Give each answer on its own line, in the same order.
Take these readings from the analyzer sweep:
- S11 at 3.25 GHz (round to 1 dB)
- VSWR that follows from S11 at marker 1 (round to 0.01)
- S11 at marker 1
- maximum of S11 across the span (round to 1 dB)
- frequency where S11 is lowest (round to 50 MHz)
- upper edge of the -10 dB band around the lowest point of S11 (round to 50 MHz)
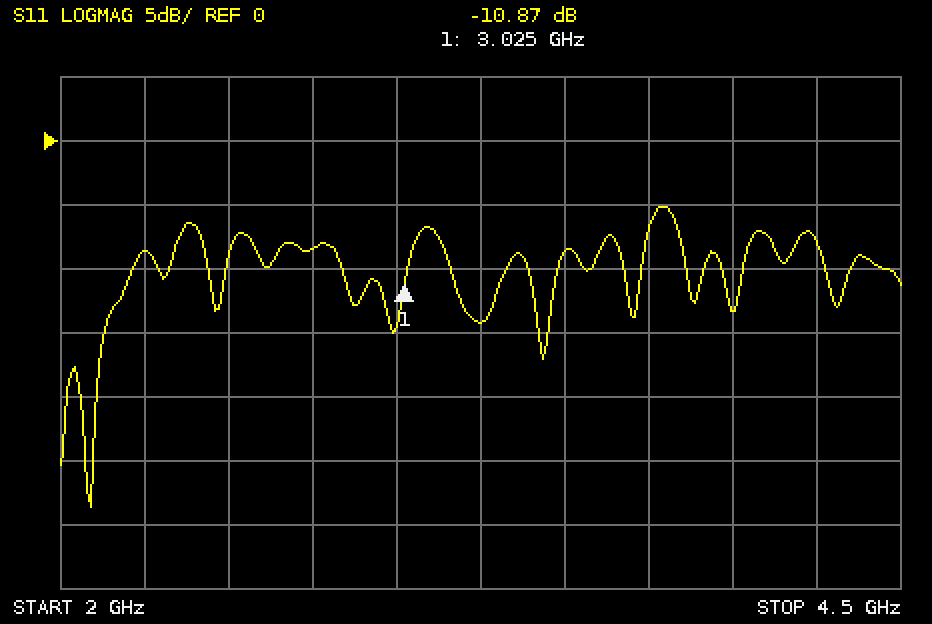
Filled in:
-14 dB
1.80
-10.87 dB
-5 dB
2.10 GHz
2.20 GHz
